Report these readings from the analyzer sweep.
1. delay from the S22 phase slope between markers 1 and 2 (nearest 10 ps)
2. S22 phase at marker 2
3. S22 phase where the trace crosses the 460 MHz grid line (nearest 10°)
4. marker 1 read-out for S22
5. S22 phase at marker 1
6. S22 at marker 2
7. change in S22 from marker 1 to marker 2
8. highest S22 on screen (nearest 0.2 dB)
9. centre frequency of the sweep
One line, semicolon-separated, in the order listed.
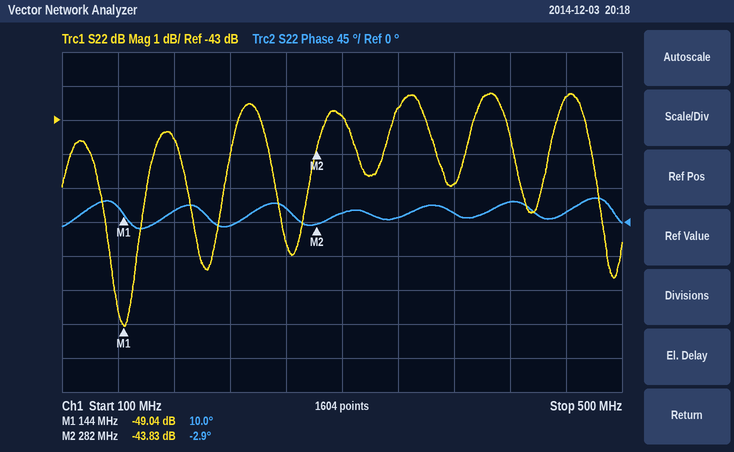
260 ps; -2.9°; 10°; -49.04 dB; 10.0°; -43.83 dB; 5.21 dB; -42.2 dB; 300 MHz
